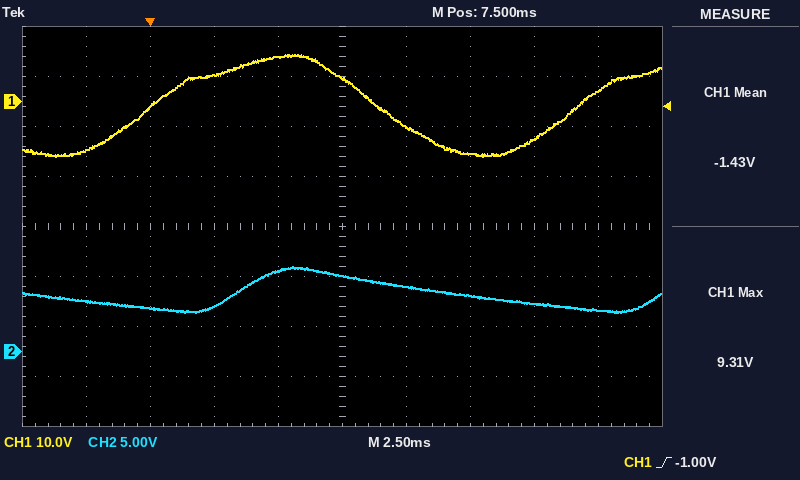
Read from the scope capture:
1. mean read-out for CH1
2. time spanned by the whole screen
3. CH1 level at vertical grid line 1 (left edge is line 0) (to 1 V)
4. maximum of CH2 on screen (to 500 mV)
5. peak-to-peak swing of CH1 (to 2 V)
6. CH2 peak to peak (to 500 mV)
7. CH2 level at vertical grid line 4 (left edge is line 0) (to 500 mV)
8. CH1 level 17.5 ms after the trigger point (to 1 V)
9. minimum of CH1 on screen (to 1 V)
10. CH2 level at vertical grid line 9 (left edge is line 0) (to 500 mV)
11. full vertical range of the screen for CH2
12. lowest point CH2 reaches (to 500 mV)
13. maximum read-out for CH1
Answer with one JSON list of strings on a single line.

["-1.43 V", "25 ms", "-10 V", "8.5 V", "20 V", "4.5 V", "8.0 V", "2 V", "-11 V", "4.0 V", "40 V", "4.0 V", "9.31 V"]
